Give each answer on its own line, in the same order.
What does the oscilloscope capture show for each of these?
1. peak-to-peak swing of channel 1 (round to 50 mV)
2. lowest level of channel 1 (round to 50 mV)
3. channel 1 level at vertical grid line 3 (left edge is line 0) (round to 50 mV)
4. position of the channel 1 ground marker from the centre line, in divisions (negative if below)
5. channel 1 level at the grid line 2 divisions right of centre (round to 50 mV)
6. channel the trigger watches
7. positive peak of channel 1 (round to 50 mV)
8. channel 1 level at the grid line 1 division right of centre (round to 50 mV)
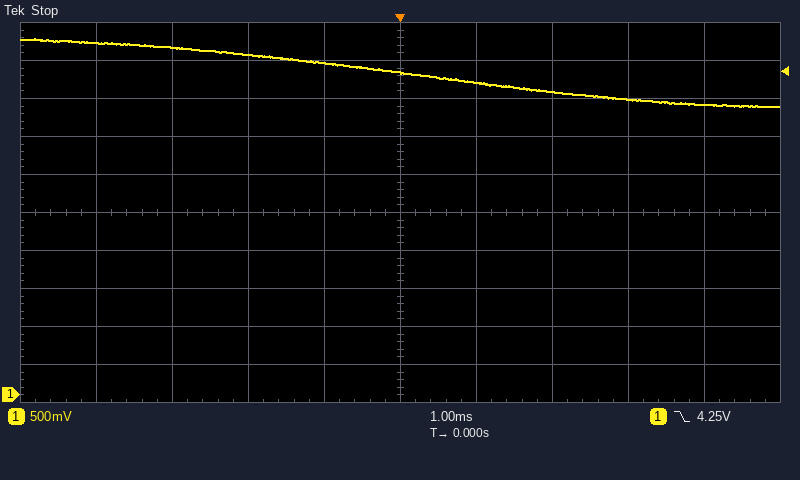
900 mV
3.80 V
4.50 V
-4.8 div
4.00 V
channel 1
4.70 V
4.10 V
